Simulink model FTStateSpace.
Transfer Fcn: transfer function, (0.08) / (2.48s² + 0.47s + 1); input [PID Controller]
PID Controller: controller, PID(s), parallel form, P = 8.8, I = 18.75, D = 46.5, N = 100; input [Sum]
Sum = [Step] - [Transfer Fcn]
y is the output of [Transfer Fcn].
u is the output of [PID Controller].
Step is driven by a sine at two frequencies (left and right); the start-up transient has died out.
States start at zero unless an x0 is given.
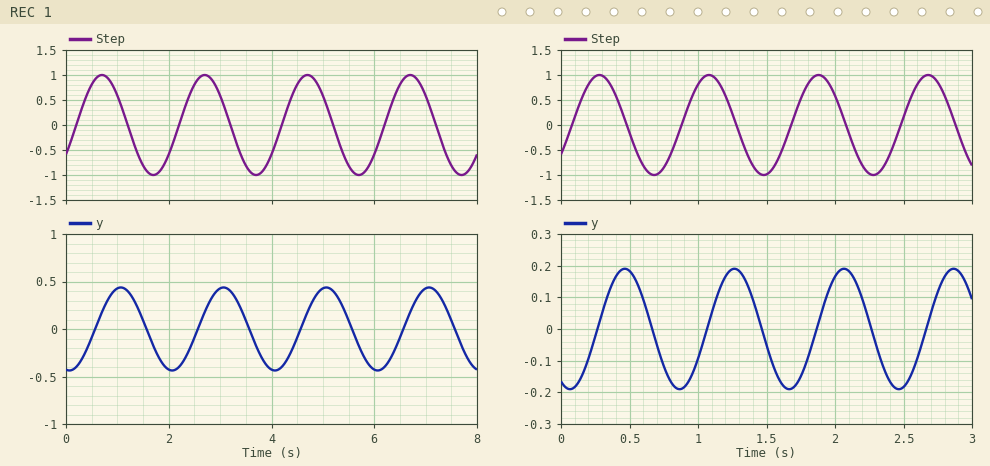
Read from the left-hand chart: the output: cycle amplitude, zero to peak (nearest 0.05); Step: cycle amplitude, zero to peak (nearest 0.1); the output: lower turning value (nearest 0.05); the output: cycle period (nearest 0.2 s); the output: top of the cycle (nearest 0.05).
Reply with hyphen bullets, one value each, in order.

- 0.45
- 1.0
- -0.45
- 2.0 s
- 0.45
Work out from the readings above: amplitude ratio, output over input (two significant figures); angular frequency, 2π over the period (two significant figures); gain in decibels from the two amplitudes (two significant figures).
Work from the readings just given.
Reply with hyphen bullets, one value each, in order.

- 0.45
- 3.1 rad/s
- -6.9 dB
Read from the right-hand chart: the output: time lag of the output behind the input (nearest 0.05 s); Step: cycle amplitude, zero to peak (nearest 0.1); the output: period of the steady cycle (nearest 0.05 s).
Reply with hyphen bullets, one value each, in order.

- 0.20 s
- 1.0
- 0.80 s
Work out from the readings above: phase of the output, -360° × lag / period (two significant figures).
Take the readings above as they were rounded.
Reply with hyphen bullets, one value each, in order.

- -90°
